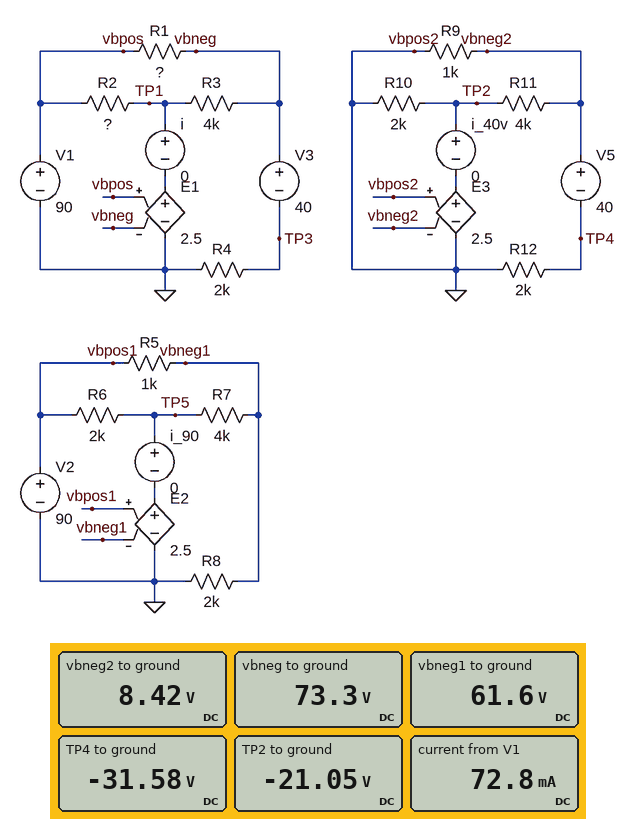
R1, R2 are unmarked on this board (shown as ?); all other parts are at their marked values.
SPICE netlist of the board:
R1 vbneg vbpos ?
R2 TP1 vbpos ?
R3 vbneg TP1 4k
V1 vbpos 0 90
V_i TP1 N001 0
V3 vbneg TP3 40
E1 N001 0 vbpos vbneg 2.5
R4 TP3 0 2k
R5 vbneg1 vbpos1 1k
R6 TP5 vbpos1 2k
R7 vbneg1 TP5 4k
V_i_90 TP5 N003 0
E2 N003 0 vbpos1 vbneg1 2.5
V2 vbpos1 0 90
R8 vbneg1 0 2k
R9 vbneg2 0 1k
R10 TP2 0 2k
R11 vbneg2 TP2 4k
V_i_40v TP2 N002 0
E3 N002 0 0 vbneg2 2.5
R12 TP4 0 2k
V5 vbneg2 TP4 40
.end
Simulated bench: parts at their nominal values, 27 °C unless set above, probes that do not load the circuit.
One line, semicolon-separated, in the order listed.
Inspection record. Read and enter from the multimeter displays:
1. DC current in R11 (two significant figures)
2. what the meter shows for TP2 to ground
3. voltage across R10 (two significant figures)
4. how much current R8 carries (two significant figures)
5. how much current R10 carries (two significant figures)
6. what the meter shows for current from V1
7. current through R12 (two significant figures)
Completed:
7.4 mA; -21.05 V; 21 V; 31 mA; 11 mA; 72.8 mA; 16 mA
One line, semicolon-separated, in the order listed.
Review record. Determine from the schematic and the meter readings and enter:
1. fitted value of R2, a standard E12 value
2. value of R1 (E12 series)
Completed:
1 kΩ; 680 Ω
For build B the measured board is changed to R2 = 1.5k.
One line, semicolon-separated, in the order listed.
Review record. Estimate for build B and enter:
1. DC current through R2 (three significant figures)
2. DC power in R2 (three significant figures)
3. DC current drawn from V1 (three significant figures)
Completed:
32.2 mA; 1.55 W; 56.7 mA
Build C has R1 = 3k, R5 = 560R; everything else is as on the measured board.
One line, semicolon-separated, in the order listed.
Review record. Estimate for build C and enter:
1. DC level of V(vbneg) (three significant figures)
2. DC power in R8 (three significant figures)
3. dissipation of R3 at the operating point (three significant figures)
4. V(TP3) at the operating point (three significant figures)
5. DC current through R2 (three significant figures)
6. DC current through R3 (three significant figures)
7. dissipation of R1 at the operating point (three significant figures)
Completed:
62.2 V; 2.36 W; 13.4 mW; 22.2 V; 20.5 mA; 1.83 mA; 258 mW
